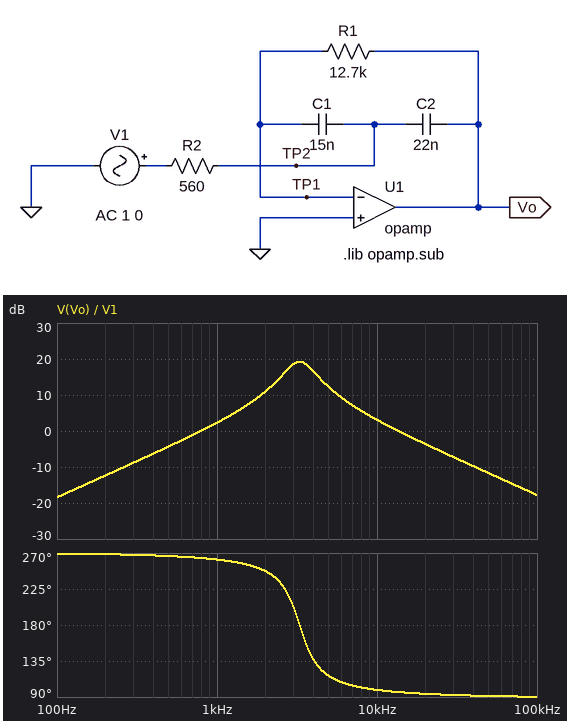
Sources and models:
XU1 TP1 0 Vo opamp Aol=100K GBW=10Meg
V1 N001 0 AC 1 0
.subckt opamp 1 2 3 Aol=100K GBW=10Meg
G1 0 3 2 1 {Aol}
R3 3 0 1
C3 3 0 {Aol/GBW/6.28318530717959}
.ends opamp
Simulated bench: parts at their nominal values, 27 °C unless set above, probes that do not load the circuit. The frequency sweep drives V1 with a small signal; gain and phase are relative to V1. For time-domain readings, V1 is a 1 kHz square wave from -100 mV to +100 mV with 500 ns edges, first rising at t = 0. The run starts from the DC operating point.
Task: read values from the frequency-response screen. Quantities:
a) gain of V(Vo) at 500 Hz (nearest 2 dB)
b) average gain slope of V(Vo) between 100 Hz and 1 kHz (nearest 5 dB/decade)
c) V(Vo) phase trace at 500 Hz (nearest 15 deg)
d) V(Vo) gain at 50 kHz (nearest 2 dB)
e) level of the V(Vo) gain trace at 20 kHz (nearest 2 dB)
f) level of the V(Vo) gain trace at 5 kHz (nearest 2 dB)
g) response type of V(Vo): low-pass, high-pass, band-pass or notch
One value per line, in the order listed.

-4 dB
20 dB/decade
270 deg
-12 dB
-4 dB
12 dB
band-pass
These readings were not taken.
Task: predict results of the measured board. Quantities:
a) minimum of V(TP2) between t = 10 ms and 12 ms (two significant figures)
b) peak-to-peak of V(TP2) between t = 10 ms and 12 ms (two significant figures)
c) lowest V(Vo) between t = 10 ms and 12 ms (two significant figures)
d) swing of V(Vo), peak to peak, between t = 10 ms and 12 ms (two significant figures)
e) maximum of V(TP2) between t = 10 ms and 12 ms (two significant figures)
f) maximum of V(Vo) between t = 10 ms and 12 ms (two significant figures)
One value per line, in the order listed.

-210 mV
420 mV
-650 mV
1.3 V
210 mV
650 mV
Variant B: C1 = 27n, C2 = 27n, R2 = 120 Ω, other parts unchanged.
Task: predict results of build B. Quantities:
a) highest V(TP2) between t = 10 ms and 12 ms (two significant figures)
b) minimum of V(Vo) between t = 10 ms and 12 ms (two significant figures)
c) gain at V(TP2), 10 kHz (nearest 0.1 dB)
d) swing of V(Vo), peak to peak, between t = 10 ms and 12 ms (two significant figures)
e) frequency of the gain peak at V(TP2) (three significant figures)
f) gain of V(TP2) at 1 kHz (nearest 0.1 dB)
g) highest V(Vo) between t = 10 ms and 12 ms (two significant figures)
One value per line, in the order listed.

270 mV
-2.0 V
-10.9 dB
4.1 V
4.72 kHz
0.4 dB
2.0 V
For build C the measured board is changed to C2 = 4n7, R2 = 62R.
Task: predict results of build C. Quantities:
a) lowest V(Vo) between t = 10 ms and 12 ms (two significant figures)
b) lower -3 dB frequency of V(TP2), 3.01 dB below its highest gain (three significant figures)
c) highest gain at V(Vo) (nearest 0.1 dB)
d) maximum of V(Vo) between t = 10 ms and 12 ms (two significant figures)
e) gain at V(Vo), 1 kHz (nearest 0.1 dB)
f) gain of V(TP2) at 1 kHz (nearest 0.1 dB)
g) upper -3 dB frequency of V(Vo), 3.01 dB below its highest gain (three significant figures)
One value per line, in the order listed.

-4.4 V
18.9 kHz
43.8 dB
4.4 V
1.6 dB
0 dB
22.5 kHz
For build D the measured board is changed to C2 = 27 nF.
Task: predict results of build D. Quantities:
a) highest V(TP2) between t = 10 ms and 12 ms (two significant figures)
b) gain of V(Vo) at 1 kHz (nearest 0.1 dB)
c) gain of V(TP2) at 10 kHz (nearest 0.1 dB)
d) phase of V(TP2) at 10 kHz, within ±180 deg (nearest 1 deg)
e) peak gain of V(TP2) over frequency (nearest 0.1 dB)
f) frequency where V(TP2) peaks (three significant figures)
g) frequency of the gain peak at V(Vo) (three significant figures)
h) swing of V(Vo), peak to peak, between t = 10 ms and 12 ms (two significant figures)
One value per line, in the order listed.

210 mV
2.5 dB
-20.5 dB
-172 deg
7.4 dB
2.82 kHz
2.96 kHz
1.2 V
